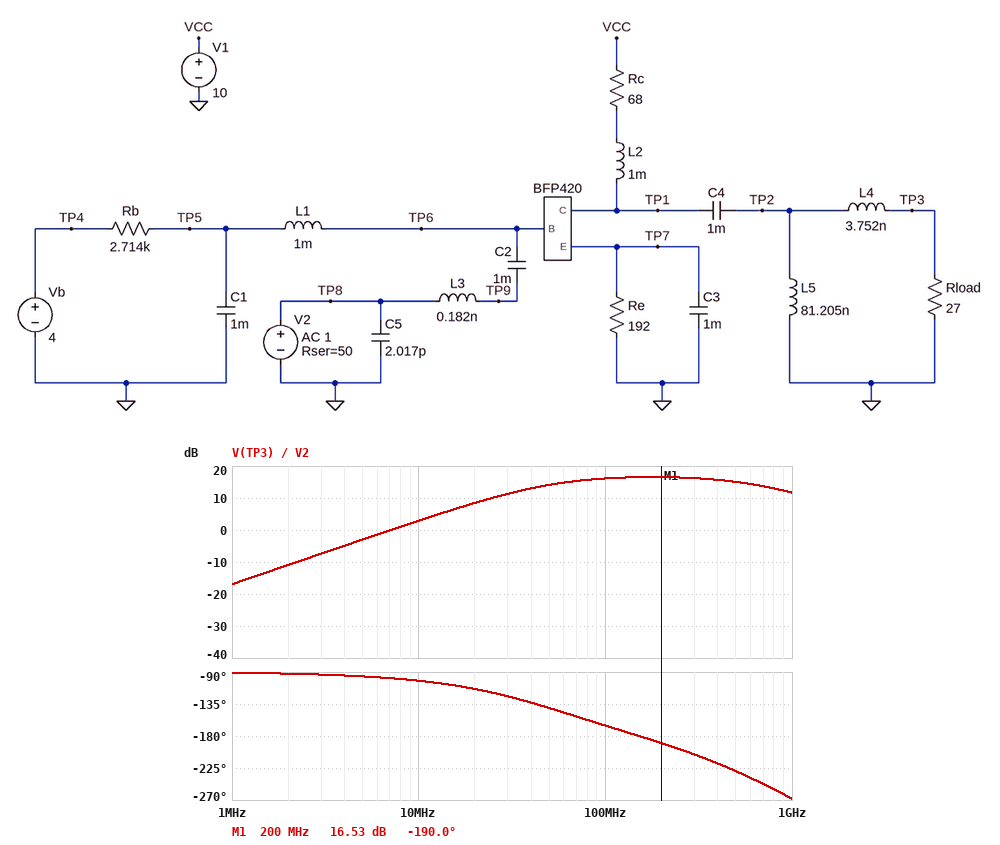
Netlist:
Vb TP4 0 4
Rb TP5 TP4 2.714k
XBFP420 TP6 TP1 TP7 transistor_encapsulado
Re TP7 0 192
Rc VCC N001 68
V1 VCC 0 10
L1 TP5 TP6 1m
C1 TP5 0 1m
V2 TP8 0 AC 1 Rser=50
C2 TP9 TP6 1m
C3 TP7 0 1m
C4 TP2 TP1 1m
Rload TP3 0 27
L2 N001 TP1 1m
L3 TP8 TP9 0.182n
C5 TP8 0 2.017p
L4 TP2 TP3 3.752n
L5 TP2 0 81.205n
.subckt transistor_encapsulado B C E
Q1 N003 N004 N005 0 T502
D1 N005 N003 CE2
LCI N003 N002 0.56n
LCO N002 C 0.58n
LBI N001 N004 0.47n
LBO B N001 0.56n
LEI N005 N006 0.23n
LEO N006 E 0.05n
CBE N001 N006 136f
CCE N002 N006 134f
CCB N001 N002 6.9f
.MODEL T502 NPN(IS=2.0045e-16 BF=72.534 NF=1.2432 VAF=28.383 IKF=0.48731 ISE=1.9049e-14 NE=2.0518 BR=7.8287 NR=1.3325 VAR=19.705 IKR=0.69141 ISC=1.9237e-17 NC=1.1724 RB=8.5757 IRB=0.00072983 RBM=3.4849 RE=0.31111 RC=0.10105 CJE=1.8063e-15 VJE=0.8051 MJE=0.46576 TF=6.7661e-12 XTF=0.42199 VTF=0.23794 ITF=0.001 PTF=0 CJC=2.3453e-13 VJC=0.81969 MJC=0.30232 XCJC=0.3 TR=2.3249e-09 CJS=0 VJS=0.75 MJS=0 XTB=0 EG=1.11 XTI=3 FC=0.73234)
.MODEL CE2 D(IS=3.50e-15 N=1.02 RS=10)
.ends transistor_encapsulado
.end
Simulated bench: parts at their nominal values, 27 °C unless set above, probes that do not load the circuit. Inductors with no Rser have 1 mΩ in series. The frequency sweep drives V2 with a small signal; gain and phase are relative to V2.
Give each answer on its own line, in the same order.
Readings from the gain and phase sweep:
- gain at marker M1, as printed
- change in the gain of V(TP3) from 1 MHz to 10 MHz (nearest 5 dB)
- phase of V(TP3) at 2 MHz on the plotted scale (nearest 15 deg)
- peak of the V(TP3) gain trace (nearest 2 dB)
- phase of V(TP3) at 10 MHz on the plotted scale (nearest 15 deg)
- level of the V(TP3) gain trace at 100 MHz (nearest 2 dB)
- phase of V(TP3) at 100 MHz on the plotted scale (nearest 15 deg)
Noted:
16.53 dB
20 dB
-90 deg
16 dB
-105 deg
16 dB
-165 deg
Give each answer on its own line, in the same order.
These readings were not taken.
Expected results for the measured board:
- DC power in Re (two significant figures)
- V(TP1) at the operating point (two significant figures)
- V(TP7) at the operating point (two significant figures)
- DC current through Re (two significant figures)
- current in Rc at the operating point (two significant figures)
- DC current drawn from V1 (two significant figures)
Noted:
33 mW
9.1 V
2.5 V
13 mA
13 mA
13 mA
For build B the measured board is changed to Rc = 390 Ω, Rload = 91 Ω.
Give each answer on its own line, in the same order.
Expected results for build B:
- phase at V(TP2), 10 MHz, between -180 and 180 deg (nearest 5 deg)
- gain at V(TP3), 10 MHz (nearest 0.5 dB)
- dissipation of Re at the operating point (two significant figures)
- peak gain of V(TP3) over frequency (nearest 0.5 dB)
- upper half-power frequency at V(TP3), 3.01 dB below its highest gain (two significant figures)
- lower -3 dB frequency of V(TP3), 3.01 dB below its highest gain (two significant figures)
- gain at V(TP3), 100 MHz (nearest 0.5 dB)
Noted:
-95 deg
2.5 dB
32 mW
25.5 dB
570 MHz
110 MHz
21.5 dB
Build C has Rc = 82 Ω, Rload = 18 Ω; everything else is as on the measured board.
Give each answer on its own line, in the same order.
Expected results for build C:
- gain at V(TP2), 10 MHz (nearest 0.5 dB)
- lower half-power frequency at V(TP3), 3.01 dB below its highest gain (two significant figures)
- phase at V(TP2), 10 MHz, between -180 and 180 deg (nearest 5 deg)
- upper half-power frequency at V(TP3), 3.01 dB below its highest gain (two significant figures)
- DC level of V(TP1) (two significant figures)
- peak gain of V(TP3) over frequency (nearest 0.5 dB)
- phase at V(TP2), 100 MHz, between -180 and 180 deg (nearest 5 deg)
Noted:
2.5 dB
31 MHz
-105 deg
750 MHz
8.9 V
13.0 dB
-165 deg
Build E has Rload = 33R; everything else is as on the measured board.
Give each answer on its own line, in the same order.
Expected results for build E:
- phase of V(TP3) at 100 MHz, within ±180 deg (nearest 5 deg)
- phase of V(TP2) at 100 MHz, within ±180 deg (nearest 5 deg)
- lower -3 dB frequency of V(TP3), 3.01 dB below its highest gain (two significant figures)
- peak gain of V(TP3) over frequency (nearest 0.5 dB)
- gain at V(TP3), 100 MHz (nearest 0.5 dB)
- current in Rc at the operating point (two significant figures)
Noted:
-160 deg
-155 deg
53 MHz
18.0 dB
17.5 dB
13 mA
